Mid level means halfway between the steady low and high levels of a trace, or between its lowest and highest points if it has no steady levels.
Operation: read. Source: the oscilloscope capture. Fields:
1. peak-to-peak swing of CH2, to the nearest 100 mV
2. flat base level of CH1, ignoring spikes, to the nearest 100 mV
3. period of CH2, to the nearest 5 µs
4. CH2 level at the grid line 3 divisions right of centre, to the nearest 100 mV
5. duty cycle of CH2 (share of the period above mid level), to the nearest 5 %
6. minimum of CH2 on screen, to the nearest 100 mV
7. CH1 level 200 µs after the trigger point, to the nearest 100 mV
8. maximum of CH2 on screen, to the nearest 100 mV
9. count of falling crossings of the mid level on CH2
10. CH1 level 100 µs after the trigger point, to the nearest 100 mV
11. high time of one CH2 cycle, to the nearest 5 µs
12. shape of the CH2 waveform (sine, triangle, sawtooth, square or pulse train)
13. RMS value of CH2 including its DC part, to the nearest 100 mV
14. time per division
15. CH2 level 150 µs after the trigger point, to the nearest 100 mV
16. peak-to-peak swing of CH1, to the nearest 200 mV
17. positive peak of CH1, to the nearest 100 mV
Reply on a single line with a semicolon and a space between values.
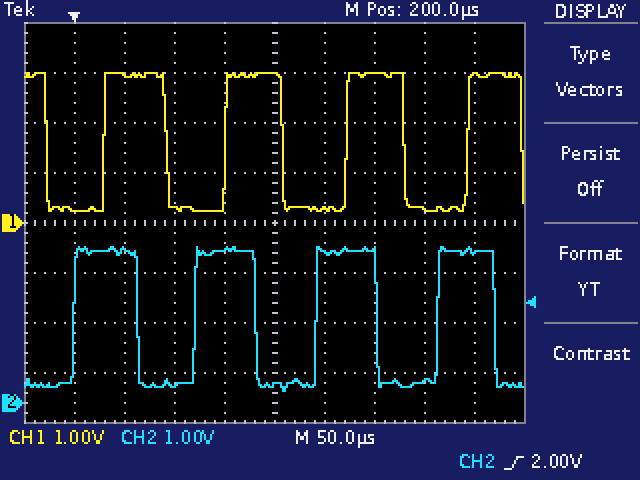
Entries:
2.9 V; 300 mV; 120 µs; 400 mV; 50 %; 200 mV; 3.0 V; 3.1 V; 4; 300 mV; 60 µs; square; 2.2 V; 50 µs; 3.1 V; 2.8 V; 3.0 V
